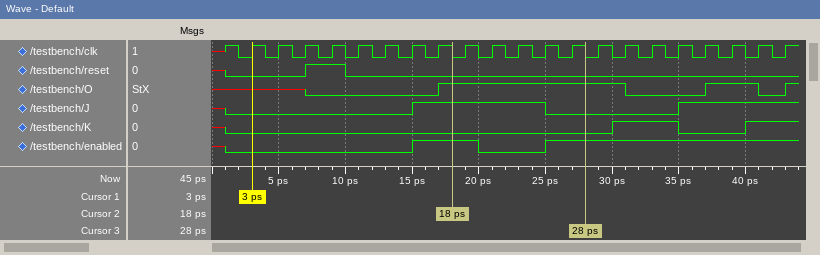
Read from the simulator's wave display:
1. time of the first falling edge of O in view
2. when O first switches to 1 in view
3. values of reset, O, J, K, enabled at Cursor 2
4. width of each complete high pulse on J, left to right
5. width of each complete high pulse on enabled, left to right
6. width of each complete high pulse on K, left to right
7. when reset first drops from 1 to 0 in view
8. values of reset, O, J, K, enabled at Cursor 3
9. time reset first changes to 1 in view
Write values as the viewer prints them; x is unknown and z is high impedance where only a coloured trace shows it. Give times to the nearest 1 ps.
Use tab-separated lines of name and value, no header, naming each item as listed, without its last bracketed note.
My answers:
time of the first falling edge of O in view	31 ps
when O first switches to 1 in view	17 ps
values of reset, O, J, K, enabled at Cursor 2	reset=0, O=1, J=1, K=0, enabled=1
width of each complete high pulse on J, left to right	10 ps
width of each complete high pulse on enabled, left to right	5 ps
width of each complete high pulse on K, left to right	5 ps
when reset first drops from 1 to 0 in view	10 ps
values of reset, O, J, K, enabled at Cursor 3	reset=0, O=1, J=0, K=0, enabled=1
time reset first changes to 1 in view	7 ps
